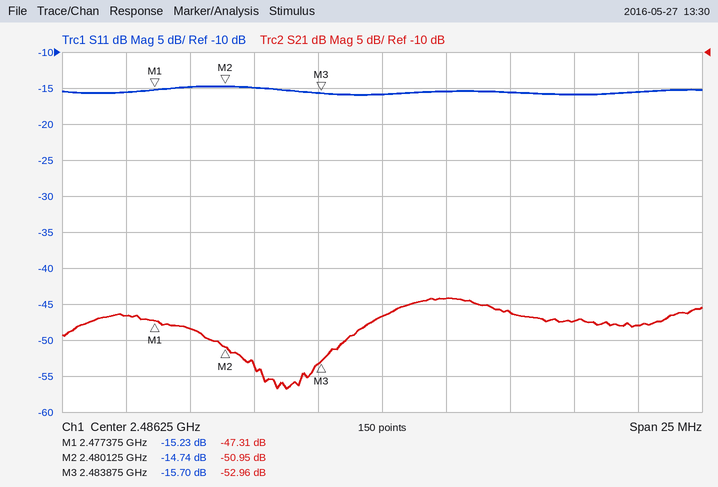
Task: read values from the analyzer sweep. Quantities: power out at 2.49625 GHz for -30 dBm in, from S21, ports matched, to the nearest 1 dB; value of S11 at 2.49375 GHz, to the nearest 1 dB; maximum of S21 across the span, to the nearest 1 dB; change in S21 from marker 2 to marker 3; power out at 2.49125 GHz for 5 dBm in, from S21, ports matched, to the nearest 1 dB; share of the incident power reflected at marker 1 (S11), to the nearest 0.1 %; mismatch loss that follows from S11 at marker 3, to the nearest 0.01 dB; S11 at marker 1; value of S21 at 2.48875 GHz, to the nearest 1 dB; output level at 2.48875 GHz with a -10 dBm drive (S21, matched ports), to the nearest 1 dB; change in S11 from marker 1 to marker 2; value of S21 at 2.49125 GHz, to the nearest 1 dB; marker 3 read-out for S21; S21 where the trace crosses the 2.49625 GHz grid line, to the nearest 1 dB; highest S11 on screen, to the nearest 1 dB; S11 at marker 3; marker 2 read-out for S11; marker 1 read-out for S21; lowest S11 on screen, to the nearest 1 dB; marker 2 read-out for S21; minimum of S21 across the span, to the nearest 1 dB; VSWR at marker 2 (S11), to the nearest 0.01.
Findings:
-78 dBm
-16 dB
-44 dB
-2.01 dB
-41 dBm
3.0 %
0.12 dB
-15.23 dB
-44 dB
-54 dBm
0.49 dB
-46 dB
-52.96 dB
-48 dB
-15 dB
-15.70 dB
-14.74 dB
-47.31 dB
-16 dB
-50.95 dB
-57 dB
1.45
